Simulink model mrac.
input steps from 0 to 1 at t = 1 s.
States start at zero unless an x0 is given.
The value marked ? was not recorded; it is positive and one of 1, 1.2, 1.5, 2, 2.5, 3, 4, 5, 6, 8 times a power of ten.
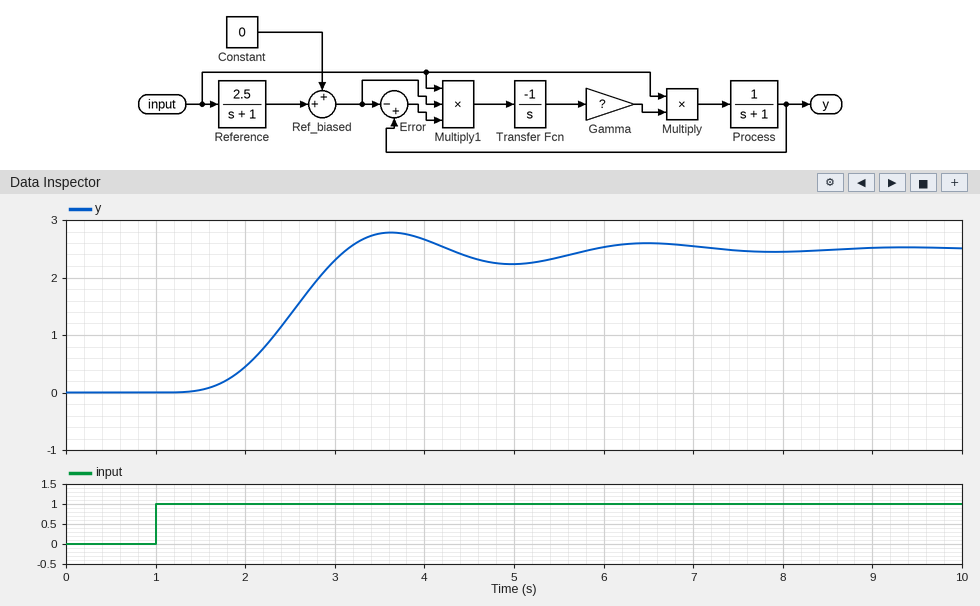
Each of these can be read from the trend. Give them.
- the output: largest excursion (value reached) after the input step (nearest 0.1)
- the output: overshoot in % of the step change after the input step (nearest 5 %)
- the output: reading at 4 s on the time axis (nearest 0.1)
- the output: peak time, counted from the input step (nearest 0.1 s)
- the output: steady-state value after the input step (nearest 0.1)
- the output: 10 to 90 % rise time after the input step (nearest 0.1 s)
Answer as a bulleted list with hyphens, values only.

- 2.8
- 10 %
- 2.7
- 2.6 s
- 2.5
- 1.1 s
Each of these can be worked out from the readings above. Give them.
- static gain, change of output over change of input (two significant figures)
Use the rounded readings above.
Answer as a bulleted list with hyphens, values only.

- 2.5
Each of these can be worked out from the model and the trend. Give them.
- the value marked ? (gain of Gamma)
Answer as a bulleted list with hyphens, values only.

- 2
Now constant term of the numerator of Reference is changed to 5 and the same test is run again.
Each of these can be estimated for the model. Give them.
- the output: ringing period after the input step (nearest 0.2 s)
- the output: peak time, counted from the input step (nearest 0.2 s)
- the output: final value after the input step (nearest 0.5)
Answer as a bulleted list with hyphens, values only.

- 2.0 s
- 2.0 s
- 5.0
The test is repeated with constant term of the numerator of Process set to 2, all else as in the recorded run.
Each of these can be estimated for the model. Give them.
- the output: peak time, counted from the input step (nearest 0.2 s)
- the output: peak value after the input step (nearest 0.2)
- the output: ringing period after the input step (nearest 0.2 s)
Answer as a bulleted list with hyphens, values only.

- 2.0 s
- 2.6
- 2.0 s
